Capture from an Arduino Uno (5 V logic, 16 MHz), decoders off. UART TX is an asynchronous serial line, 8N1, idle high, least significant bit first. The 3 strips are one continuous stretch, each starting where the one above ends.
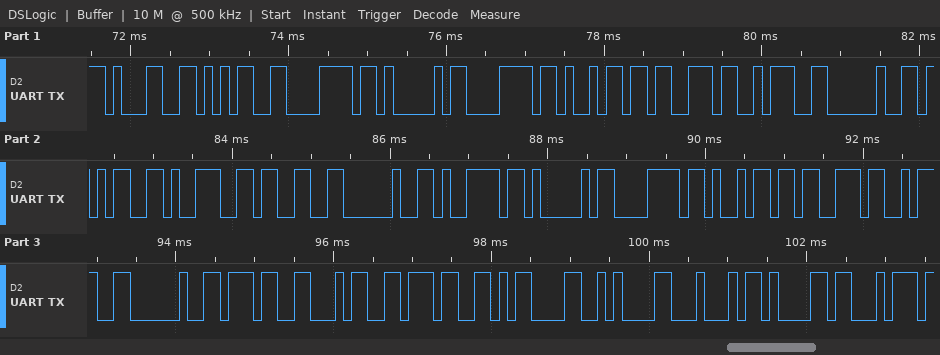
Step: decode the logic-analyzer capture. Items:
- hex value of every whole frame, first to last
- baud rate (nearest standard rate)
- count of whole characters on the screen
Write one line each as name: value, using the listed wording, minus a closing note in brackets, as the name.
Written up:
hex value of every whole frame, first to last: 31 35 78 41 78 69 73 3A 20 35 39 33 20 79 41 78 69 73 3A 20 37 34 37 0D 0A 44 61 74
baud rate: 9600 baud
count of whole characters on the screen: 28
